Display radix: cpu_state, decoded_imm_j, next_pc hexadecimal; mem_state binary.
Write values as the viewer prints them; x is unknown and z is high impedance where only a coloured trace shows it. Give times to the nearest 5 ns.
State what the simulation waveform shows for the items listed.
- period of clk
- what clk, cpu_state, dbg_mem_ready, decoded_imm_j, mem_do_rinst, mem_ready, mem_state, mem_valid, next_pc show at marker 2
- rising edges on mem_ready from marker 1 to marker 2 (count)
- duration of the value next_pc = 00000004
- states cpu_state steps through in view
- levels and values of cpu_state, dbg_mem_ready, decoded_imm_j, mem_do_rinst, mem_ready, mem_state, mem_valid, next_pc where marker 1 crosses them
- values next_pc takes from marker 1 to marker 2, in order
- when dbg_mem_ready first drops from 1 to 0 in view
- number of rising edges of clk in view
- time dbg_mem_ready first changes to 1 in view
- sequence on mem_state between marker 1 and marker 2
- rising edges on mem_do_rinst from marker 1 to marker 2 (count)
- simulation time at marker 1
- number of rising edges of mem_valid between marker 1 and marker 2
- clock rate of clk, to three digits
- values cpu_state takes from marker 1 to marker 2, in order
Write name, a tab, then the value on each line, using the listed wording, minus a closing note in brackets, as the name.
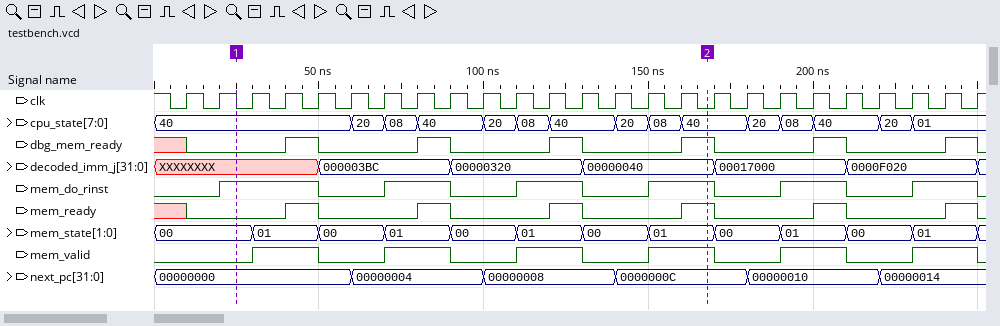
period of clk	10 ns
what clk, cpu_state, dbg_mem_ready, decoded_imm_j, mem_do_rinst, mem_ready, mem_state, mem_valid, next_pc show at marker 2	clk=0, cpu_state=40, dbg_mem_ready=1, decoded_imm_j=00000040, mem_do_rinst=1, mem_ready=1, mem_state=01, mem_valid=1, next_pc=0000000C
rising edges on mem_ready from marker 1 to marker 2	4
duration of the value next_pc = 00000004	40 ns
states cpu_state steps through in view	40, 20, 08, 40, 20, 08, 40, 20, 08, 40, 20, 08, 40, 20, 01
levels and values of cpu_state, dbg_mem_ready, decoded_imm_j, mem_do_rinst, mem_ready, mem_state, mem_valid, next_pc where marker 1 crosses them	cpu_state=40, dbg_mem_ready=0, decoded_imm_j=XXXXXXXX, mem_do_rinst=1, mem_ready=0, mem_state=00, mem_valid=0, next_pc=00000000
values next_pc takes from marker 1 to marker 2, in order	00000000, 00000004, 00000008, 0000000C
when dbg_mem_ready first drops from 1 to 0 in view	50 ns
number of rising edges of clk in view	25
time dbg_mem_ready first changes to 1 in view	40 ns
sequence on mem_state between marker 1 and marker 2	00, 01, 00, 01, 00, 01, 00, 01
rising edges on mem_do_rinst from marker 1 to marker 2	3
simulation time at marker 1	25 ns
number of rising edges of mem_valid between marker 1 and marker 2	4
clock rate of clk, to three digits	100 MHz
values cpu_state takes from marker 1 to marker 2, in order	40, 20, 08, 40, 20, 08, 40, 20, 08, 40
